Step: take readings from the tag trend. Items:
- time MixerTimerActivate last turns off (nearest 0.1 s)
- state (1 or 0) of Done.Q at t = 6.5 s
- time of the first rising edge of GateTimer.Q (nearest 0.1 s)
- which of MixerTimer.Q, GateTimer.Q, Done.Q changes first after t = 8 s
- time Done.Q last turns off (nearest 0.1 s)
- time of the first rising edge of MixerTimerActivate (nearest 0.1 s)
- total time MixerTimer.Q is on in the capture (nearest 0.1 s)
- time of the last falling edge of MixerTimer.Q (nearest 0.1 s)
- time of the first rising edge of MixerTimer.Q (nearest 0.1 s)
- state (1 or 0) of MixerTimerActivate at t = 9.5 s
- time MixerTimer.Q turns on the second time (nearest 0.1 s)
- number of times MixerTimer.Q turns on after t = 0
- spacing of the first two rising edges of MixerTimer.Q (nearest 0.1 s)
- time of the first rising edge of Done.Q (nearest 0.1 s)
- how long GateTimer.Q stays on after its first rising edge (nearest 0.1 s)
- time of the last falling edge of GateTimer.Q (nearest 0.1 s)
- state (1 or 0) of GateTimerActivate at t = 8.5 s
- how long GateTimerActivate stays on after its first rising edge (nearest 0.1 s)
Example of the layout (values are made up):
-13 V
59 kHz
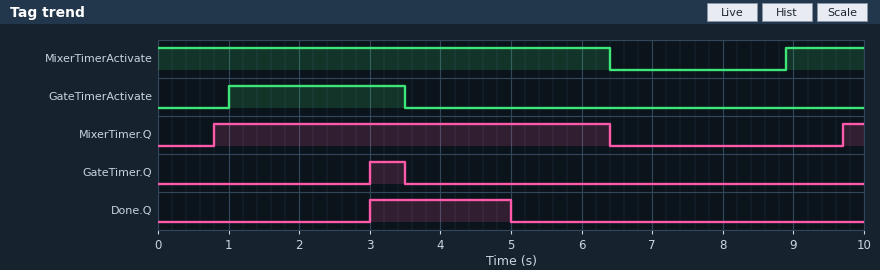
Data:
6.4 s
0
3.0 s
MixerTimer.Q
5.0 s
8.9 s
5.9 s
6.4 s
0.8 s
1
9.7 s
2
8.9 s
3.0 s
0.5 s
3.5 s
0
2.5 s
